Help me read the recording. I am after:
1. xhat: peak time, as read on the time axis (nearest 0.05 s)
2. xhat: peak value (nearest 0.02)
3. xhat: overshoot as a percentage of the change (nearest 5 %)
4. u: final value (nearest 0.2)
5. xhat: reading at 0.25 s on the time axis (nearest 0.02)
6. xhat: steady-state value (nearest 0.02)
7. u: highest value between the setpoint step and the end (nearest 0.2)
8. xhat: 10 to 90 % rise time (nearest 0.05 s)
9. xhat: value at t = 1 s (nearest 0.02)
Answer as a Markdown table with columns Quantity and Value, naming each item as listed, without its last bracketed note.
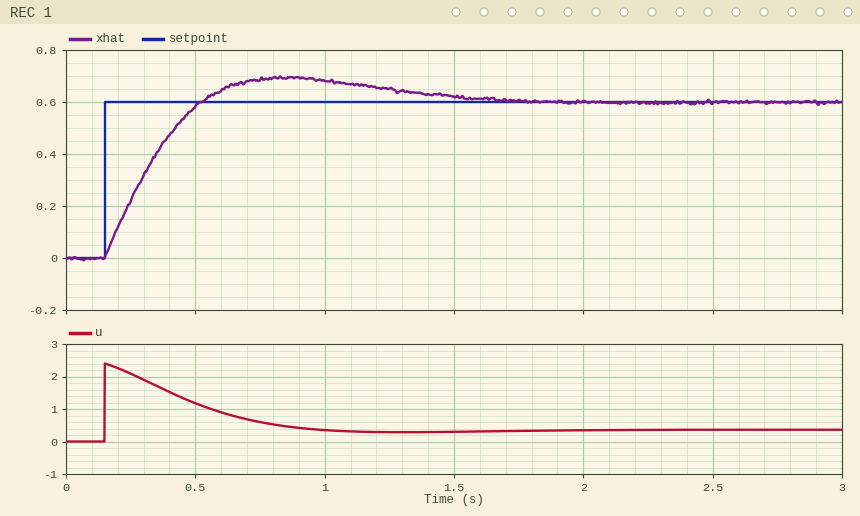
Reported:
| Quantity | Value |
|---|---|
| xhat: peak time, as read on the time axis | 0.85 s |
| xhat: peak value | 0.70 |
| xhat: overshoot as a percentage of the change | 15 % |
| u: final value | 0.4 |
| xhat: reading at 0.25 s on the time axis | 0.22 |
| xhat: steady-state value | 0.60 |
| u: highest value between the setpoint step and the end | 2.4 |
| xhat: 10 to 90 % rise time | 0.30 s |
| xhat: value at t = 1 s | 0.68 |
